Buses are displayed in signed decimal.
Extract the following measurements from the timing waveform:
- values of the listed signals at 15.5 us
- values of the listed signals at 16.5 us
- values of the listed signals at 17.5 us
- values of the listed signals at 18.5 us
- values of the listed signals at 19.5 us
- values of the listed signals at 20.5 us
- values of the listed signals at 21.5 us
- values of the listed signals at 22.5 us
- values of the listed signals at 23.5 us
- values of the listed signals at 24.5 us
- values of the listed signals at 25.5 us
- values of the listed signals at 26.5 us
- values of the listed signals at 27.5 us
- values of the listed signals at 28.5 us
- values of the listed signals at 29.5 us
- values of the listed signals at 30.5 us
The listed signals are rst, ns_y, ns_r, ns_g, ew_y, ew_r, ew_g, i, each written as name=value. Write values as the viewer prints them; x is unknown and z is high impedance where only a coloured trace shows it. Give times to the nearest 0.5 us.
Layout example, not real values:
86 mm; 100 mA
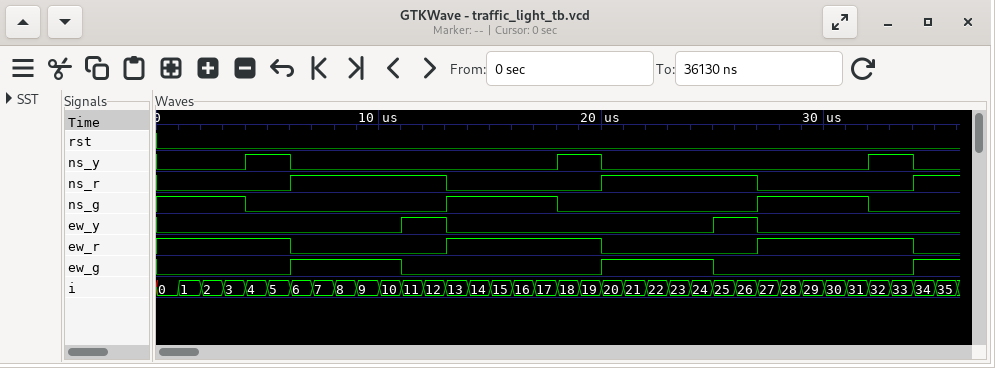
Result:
rst=0, ns_y=0, ns_r=0, ns_g=1, ew_y=0, ew_r=1, ew_g=0, i=15; rst=0, ns_y=0, ns_r=0, ns_g=1, ew_y=0, ew_r=1, ew_g=0, i=16; rst=0, ns_y=0, ns_r=0, ns_g=1, ew_y=0, ew_r=1, ew_g=0, i=17; rst=0, ns_y=1, ns_r=0, ns_g=0, ew_y=0, ew_r=1, ew_g=0, i=18; rst=0, ns_y=1, ns_r=0, ns_g=0, ew_y=0, ew_r=1, ew_g=0, i=19; rst=0, ns_y=0, ns_r=1, ns_g=0, ew_y=0, ew_r=0, ew_g=1, i=20; rst=0, ns_y=0, ns_r=1, ns_g=0, ew_y=0, ew_r=0, ew_g=1, i=21; rst=0, ns_y=0, ns_r=1, ns_g=0, ew_y=0, ew_r=0, ew_g=1, i=22; rst=0, ns_y=0, ns_r=1, ns_g=0, ew_y=0, ew_r=0, ew_g=1, i=23; rst=0, ns_y=0, ns_r=1, ns_g=0, ew_y=0, ew_r=0, ew_g=1, i=24; rst=0, ns_y=0, ns_r=1, ns_g=0, ew_y=1, ew_r=0, ew_g=0, i=25; rst=0, ns_y=0, ns_r=1, ns_g=0, ew_y=1, ew_r=0, ew_g=0, i=26; rst=0, ns_y=0, ns_r=0, ns_g=1, ew_y=0, ew_r=1, ew_g=0, i=27; rst=0, ns_y=0, ns_r=0, ns_g=1, ew_y=0, ew_r=1, ew_g=0, i=28; rst=0, ns_y=0, ns_r=0, ns_g=1, ew_y=0, ew_r=1, ew_g=0, i=29; rst=0, ns_y=0, ns_r=0, ns_g=1, ew_y=0, ew_r=1, ew_g=0, i=30
